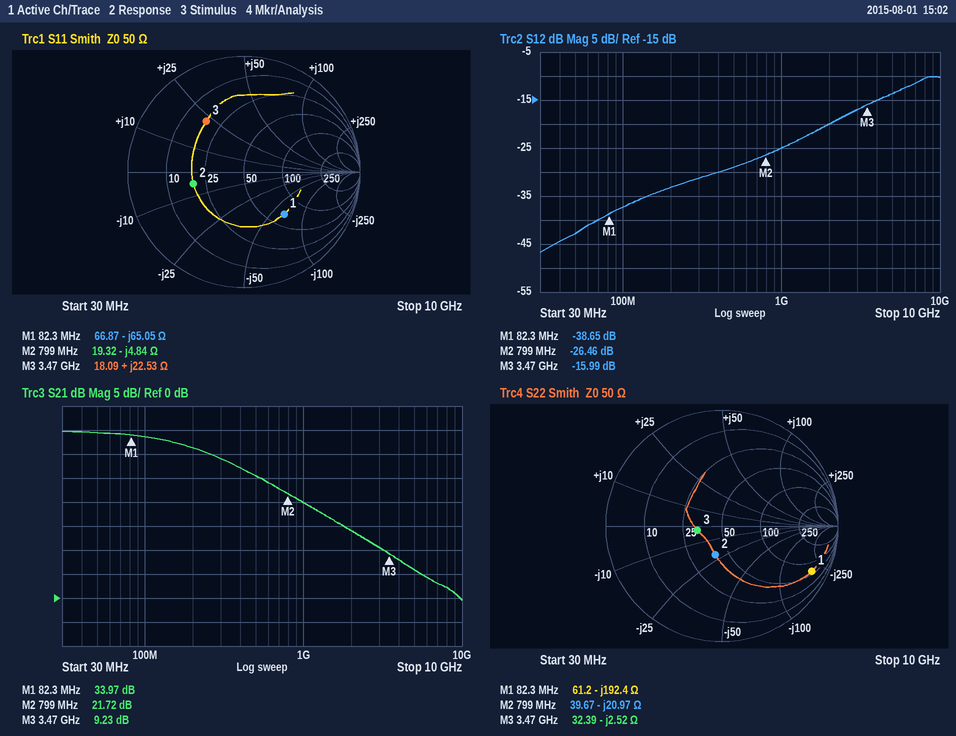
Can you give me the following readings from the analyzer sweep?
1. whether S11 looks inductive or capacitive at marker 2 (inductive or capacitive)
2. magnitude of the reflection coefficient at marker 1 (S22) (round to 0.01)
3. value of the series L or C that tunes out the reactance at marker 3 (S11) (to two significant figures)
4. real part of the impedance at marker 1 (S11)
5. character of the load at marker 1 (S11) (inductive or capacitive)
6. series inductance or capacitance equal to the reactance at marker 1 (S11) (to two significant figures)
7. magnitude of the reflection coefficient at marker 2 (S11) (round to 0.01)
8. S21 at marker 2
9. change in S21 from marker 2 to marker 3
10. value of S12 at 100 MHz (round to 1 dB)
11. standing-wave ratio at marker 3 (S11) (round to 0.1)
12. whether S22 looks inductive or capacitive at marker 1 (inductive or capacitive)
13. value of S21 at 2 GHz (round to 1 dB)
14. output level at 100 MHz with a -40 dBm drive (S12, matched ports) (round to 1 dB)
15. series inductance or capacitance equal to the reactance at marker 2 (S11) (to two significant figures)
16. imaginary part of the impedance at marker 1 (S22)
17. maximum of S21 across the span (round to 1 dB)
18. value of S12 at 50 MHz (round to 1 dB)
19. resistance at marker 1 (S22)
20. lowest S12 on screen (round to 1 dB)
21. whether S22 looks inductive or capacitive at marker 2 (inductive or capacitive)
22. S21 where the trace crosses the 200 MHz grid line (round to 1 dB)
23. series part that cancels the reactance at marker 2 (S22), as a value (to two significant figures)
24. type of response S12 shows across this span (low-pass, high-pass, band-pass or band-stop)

capacitive
0.87
2.0 pF
66.87 Ω
capacitive
30 pF
0.45
21.72 dB
-12.49 dB
-37 dB
3.4
capacitive
14 dB
-77 dBm
41 pF
-192.4 Ω
35 dB
-43 dB
61.2 Ω
-47 dB
capacitive
31 dB
4.2 nH
high-pass
